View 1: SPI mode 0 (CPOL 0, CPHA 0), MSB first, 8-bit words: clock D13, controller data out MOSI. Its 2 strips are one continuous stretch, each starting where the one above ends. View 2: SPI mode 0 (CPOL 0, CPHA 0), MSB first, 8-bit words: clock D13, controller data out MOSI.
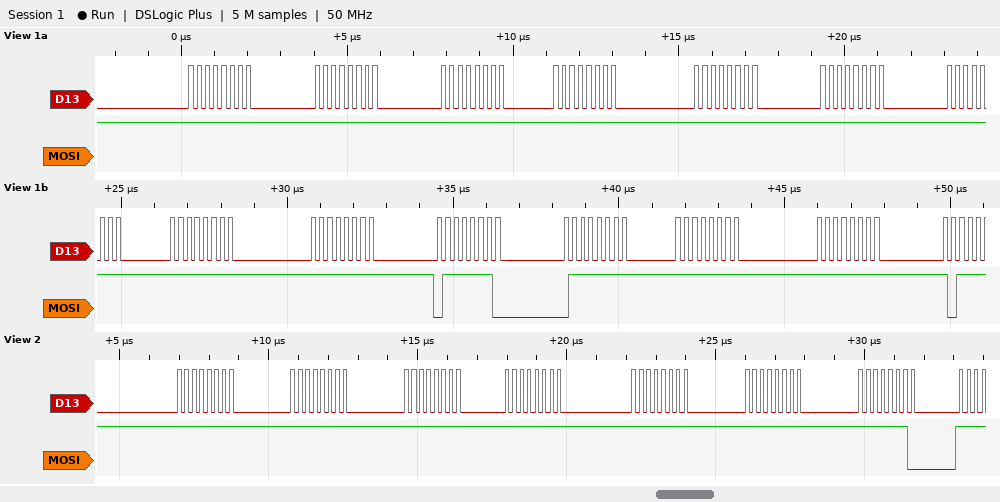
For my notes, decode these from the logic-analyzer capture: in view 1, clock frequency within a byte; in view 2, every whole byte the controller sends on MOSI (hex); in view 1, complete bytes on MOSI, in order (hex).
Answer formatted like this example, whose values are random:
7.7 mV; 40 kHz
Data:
4 MHz; FF FF FF FF FF FF FE; FF FF FF FF FF FF FF FF FF 7E 7F FF FF
